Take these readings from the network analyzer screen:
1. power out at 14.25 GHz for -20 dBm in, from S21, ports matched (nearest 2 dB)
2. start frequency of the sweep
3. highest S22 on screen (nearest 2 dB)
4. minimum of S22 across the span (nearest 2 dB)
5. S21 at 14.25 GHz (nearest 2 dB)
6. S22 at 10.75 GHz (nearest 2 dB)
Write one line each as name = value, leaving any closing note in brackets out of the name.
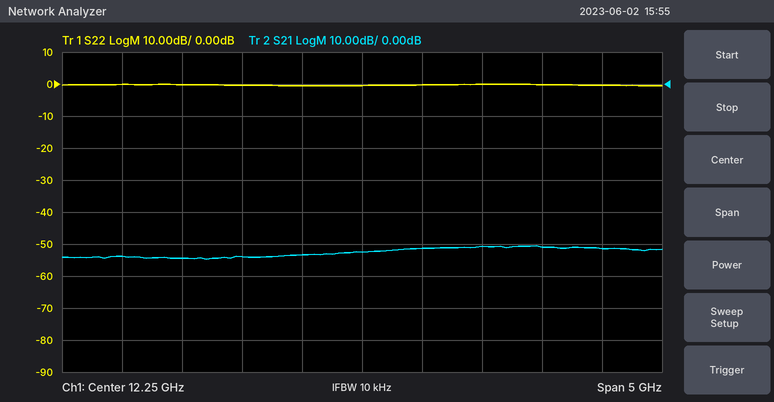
power out at 14.25 GHz for -20 dBm in, from S21, ports matched = -72 dBm
start frequency of the sweep = 9.75 GHz
highest S22 on screen = 0 dB
minimum of S22 across the span = 0 dB
S21 at 14.25 GHz = -52 dB
S22 at 10.75 GHz = 0 dB
